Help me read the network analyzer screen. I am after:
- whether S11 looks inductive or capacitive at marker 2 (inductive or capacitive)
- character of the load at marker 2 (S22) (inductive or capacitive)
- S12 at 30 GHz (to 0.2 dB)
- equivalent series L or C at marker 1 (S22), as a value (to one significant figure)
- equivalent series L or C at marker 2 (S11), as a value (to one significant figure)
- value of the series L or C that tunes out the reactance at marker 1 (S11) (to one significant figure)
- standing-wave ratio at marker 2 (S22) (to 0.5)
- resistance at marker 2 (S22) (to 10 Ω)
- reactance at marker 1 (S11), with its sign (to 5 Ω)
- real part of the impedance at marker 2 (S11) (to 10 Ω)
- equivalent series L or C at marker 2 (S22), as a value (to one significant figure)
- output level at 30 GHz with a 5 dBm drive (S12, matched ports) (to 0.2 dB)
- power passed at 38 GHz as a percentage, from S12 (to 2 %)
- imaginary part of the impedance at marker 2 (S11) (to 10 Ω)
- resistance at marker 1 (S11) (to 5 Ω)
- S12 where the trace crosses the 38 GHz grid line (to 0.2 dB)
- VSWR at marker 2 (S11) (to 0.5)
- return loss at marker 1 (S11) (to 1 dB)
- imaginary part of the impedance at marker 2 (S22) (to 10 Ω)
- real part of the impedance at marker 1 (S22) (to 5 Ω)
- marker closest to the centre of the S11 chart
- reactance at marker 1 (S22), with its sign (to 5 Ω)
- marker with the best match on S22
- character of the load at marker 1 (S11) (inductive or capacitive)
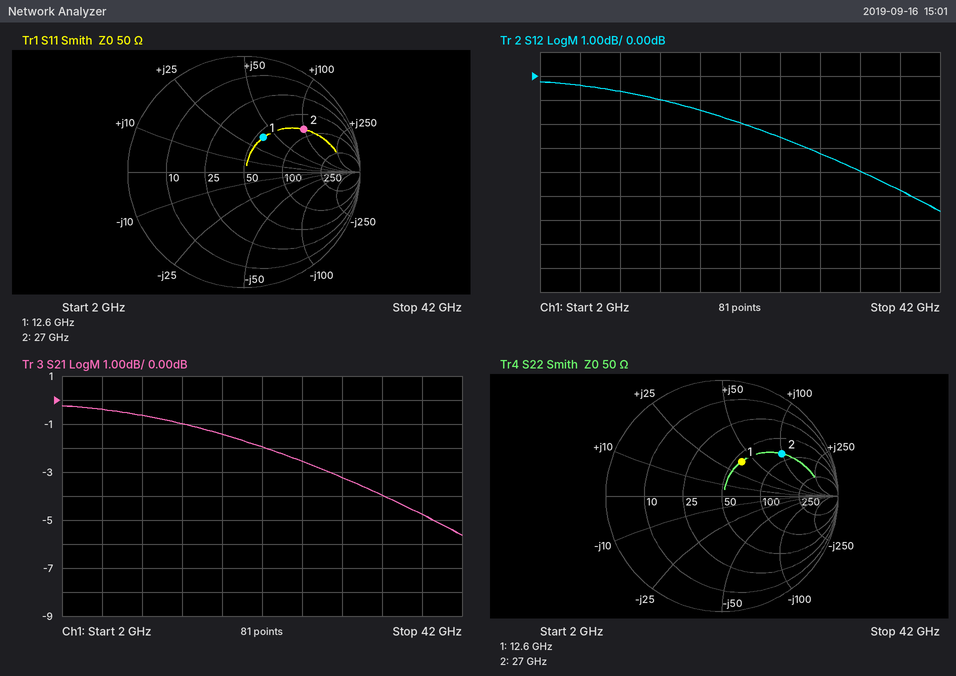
inductive
inductive
-3.2 dB
500 pH
600 pH
300 fF
4.5
80 Ω
+40 Ω
80 Ω
600 pH
1.8 dBm
34 %
+100 Ω
55 Ω
-4.8 dB
4.5
9 dB
+100 Ω
55 Ω
marker 1
+40 Ω
marker 1
inductive
